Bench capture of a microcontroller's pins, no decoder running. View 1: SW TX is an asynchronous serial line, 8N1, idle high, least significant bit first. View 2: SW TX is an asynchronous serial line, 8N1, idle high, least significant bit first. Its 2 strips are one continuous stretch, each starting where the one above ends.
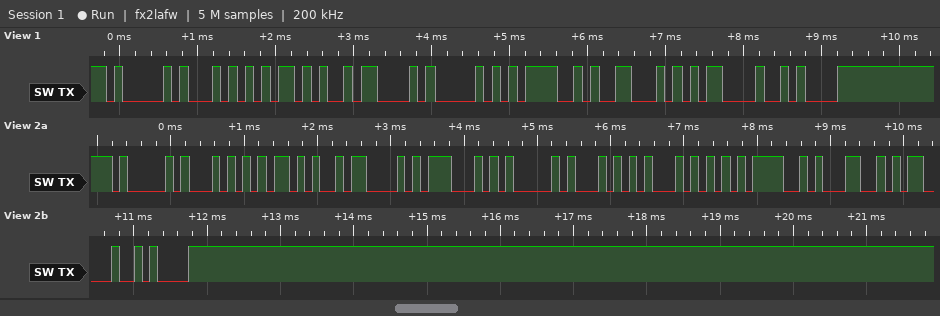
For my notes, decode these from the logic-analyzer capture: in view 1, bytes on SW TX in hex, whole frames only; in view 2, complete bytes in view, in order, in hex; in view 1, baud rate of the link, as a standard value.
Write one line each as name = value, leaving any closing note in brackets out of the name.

in view 1, bytes on SW TX in hex, whole frames only = 41 54 2B 43 50 4F 46 0D 0A
in view 2, complete bytes in view, in order, in hex = 0x41 0x54 0x2B 0x43 0x47 0x41 0x54 0x54 0x3D 0x31 0x0D 0x0A
in view 1, baud rate of the link, as a standard value = 9600 baud
